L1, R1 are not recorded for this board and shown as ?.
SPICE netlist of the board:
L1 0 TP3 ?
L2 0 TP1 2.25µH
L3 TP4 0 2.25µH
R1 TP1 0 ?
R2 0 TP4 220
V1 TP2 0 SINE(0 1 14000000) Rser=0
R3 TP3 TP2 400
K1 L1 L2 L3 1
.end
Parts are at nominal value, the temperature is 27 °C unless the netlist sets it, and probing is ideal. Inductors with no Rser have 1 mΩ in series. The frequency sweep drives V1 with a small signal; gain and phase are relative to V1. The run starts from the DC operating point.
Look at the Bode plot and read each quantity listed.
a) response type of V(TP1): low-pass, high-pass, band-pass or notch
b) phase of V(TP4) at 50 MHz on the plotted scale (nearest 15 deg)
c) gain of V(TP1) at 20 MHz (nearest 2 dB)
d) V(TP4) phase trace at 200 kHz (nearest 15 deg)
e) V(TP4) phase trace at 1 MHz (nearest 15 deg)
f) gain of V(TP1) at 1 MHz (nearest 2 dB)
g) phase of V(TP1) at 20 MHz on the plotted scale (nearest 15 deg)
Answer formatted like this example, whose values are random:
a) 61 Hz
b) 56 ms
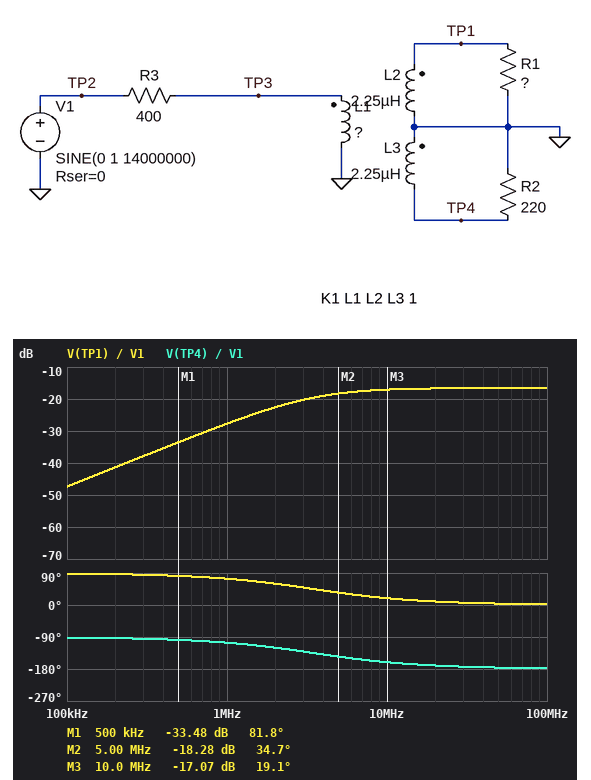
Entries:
a) high-pass
b) -180 deg
c) -16 dB
d) -90 deg
e) -105 deg
f) -28 dB
g) 15 deg
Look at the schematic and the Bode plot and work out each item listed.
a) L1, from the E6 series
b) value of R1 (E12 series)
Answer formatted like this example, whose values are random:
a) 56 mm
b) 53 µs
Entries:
a) 3.3 µH
b) 82 Ω
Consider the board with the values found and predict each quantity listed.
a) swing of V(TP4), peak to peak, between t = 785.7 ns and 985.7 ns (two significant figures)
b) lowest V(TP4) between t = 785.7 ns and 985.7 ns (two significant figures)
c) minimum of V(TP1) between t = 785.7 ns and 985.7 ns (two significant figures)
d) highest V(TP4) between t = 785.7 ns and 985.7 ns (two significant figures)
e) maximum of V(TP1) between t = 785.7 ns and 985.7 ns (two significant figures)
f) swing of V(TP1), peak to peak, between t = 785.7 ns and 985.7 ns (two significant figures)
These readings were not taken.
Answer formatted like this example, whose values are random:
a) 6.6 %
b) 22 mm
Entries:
a) 290 mV
b) -140 mV
c) -140 mV
d) 140 mV
e) 140 mV
f) 290 mV
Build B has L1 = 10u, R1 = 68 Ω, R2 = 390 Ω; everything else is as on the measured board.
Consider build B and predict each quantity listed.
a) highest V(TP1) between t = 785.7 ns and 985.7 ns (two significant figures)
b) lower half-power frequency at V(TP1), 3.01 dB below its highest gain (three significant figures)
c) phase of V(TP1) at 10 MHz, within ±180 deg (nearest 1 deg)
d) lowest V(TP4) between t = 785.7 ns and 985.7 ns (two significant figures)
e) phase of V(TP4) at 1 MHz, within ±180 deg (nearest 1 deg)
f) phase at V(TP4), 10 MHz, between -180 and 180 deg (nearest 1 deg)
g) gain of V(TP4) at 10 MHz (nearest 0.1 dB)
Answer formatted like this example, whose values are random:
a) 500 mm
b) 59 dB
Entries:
a) 180 mV
b) 2.49 MHz
c) 14 deg
d) -180 mV
e) -112 deg
f) -166 deg
g) -14.9 dB
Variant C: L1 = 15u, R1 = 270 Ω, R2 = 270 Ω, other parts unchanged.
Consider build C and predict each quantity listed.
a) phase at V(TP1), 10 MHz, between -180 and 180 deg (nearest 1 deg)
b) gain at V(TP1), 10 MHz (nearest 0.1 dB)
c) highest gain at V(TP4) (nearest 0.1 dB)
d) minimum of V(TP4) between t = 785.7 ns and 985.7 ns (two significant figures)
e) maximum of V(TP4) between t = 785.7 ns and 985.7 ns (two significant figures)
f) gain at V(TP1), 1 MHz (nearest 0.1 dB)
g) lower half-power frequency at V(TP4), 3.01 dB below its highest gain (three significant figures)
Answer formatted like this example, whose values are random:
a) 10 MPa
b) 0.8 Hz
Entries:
a) 16 deg
b) -11.8 dB
c) -11.4 dB
d) -260 mV
e) 260 mV
f) -21.3 dB
g) 2.94 MHz
